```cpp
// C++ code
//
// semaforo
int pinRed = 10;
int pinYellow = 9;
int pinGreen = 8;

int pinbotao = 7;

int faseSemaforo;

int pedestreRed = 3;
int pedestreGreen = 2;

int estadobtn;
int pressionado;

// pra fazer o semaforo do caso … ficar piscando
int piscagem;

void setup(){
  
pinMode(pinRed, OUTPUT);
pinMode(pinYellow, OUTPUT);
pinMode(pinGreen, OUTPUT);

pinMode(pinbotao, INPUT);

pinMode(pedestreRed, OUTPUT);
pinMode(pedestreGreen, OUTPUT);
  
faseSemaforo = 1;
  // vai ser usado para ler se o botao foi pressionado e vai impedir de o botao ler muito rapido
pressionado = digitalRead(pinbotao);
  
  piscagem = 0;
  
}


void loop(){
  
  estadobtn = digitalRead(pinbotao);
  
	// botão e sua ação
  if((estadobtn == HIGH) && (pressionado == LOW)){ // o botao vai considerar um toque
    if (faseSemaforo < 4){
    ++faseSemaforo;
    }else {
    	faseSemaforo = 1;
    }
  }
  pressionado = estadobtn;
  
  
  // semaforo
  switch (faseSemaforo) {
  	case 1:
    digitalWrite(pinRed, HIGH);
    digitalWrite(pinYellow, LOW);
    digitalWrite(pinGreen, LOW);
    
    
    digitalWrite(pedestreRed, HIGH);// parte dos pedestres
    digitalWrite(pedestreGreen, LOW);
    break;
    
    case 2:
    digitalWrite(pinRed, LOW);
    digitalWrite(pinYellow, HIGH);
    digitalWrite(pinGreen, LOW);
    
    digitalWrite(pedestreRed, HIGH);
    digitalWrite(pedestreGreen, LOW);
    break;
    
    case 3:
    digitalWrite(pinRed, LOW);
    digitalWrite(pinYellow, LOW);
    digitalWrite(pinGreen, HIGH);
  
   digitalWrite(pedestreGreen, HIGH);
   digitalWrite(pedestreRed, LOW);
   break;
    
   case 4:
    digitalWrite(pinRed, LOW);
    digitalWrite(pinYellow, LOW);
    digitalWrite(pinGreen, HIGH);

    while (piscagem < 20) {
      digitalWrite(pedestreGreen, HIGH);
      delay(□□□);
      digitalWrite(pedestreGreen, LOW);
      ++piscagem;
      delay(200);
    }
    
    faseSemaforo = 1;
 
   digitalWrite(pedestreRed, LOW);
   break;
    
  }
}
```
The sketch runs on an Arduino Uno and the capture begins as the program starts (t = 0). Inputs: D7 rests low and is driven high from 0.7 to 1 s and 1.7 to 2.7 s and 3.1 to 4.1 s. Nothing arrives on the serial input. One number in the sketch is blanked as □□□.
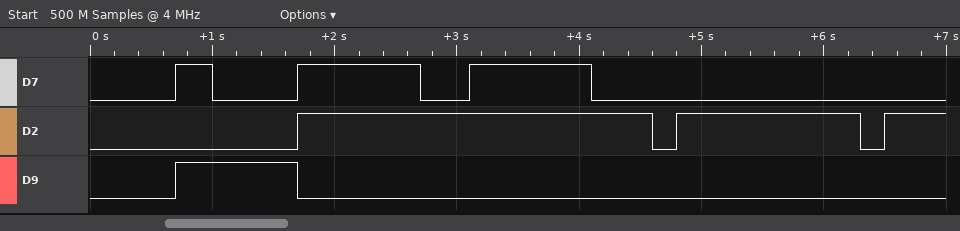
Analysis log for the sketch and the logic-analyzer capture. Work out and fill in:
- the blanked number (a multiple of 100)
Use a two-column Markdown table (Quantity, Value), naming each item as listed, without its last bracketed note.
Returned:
| Quantity | Value |
|---|---|
| the blanked number | 1500 |
